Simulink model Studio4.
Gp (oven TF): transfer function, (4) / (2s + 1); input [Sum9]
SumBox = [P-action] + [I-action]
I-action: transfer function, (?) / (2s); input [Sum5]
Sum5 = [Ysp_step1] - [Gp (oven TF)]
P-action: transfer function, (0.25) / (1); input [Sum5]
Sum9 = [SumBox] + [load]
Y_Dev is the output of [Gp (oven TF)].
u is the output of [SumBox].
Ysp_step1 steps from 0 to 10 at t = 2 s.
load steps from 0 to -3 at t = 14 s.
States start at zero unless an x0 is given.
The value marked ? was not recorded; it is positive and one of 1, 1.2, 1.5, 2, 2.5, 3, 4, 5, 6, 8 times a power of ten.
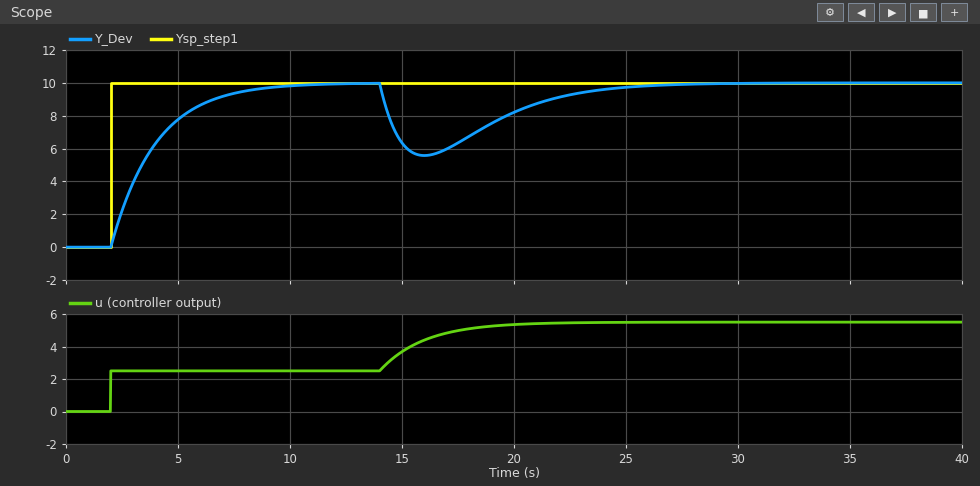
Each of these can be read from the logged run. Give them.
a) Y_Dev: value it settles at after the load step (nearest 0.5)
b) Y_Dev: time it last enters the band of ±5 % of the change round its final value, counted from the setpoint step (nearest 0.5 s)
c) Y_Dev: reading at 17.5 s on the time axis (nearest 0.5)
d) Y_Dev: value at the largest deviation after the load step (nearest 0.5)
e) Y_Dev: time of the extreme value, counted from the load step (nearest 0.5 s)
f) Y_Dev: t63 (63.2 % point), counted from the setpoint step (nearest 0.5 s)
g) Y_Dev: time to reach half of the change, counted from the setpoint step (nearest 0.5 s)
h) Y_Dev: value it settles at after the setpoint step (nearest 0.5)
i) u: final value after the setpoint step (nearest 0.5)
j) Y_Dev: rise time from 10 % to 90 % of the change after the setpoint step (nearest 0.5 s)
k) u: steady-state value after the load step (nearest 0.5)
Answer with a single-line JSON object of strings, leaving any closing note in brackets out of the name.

{"Y_Dev: value it settles at after the load step": "10.0", "Y_Dev: time it last enters the band of ±5 % of the change round its final value, counted from the setpoint step": "6.0 s", "Y_Dev: reading at 17.5 s on the time axis": "6.5", "Y_Dev: value at the largest deviation after the load step": "5.5", "Y_Dev: time of the extreme value, counted from the load step": "2.0 s", "Y_Dev: t63 (63.2 % point), counted from the setpoint step": "2.0 s", "Y_Dev: time to reach half of the change, counted from the setpoint step": "1.5 s", "Y_Dev: value it settles at after the setpoint step": "10.0", "u: final value after the setpoint step": "2.5", "Y_Dev: rise time from 10 % to 90 % of the change after the setpoint step": "4.5 s", "u: steady-state value after the load step": "5.5"}
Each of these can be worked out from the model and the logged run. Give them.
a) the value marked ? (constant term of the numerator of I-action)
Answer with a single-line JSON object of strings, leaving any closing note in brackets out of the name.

{"the value marked ?": "0.25"}
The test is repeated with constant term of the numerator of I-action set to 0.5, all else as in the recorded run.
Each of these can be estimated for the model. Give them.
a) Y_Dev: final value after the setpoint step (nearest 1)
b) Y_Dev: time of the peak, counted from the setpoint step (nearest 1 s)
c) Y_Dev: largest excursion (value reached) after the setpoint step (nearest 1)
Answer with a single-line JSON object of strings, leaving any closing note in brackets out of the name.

{"Y_Dev: final value after the setpoint step": "10", "Y_Dev: time of the peak, counted from the setpoint step": "5 s", "Y_Dev: largest excursion (value reached) after the setpoint step": "11"}
